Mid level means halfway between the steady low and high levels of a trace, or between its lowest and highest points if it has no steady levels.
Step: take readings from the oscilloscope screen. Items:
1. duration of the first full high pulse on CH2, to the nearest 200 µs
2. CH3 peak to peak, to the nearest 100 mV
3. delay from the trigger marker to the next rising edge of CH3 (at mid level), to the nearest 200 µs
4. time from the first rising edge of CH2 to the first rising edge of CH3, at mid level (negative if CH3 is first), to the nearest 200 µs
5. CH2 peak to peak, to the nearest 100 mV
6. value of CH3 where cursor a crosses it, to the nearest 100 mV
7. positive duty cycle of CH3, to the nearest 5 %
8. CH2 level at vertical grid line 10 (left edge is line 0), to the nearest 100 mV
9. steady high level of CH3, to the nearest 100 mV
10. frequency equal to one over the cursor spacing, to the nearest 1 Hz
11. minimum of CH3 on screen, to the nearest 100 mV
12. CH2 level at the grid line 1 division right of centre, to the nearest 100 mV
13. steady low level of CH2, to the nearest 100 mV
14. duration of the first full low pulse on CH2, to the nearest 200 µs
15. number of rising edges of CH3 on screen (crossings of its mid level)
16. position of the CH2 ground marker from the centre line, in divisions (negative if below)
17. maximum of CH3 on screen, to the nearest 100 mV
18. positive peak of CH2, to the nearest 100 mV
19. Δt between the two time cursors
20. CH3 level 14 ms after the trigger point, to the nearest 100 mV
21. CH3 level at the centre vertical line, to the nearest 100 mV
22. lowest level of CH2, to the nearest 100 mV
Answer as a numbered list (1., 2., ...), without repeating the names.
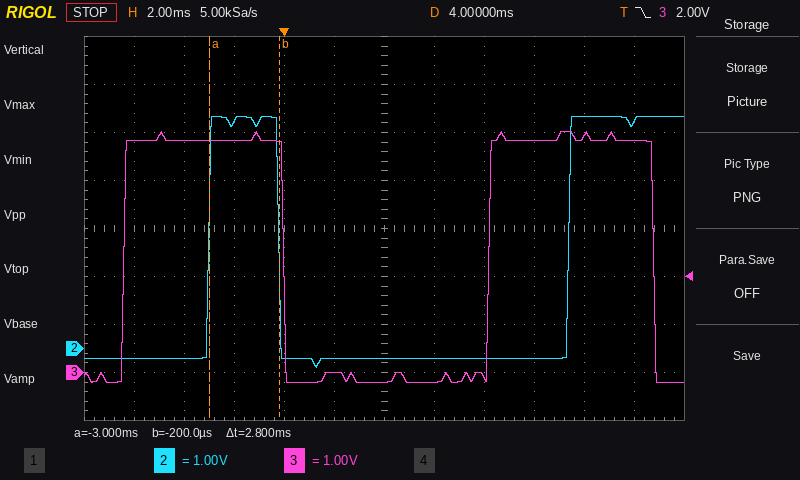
1. 2.8 ms
2. 5.2 V
3. 8.2 ms
4. -3.4 ms
5. 5.2 V
6. 4.8 V
7. 45 %
8. 4.8 V
9. 4.8 V
10. 357 Hz
11. -200 mV
12. -200 mV
13. -200 mV
14. 11.6 ms
15. 2
16. -2.5 div
17. 5.0 V
18. 4.8 V
19. 2.8 ms
20. 4.8 V
21. -200 mV
22. -400 mV
